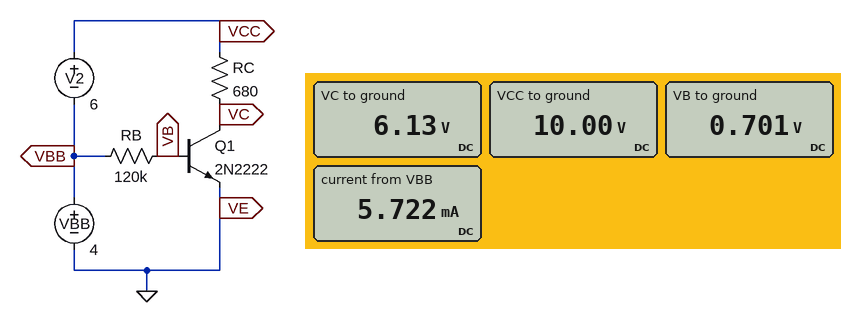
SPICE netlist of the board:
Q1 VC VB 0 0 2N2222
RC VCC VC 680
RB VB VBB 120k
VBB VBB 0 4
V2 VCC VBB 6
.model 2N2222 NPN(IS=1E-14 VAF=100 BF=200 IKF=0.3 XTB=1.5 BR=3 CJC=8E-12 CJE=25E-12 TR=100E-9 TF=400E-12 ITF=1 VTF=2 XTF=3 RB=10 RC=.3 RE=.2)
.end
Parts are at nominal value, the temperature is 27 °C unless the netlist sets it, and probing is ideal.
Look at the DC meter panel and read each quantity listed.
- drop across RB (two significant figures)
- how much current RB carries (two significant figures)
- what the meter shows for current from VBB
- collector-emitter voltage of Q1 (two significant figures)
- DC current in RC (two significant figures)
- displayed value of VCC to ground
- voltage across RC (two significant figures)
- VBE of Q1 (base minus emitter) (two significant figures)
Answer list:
3.3 V
27 µA
5.722 mA
6.1 V
5.7 mA
10.00 V
3.9 V
700 mV
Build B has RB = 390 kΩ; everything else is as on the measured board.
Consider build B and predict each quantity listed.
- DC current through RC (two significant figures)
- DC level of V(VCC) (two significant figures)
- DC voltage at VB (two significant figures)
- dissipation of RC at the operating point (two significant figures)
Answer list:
1.8 mA
10 V
670 mV
2.3 mW
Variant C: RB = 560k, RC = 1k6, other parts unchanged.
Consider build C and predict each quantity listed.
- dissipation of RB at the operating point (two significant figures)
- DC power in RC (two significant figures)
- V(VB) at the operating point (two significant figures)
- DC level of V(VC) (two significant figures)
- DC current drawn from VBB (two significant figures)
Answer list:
20 µW
2.6 mW
660 mV
8.0 V
1.3 mA
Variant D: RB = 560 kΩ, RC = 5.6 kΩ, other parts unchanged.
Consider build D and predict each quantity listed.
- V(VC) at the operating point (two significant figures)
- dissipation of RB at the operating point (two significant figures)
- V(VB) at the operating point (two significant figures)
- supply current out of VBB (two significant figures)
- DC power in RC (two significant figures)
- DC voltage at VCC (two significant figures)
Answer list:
3.2 V
20 µW
660 mV
1.2 mA
8.3 mW
10 V
